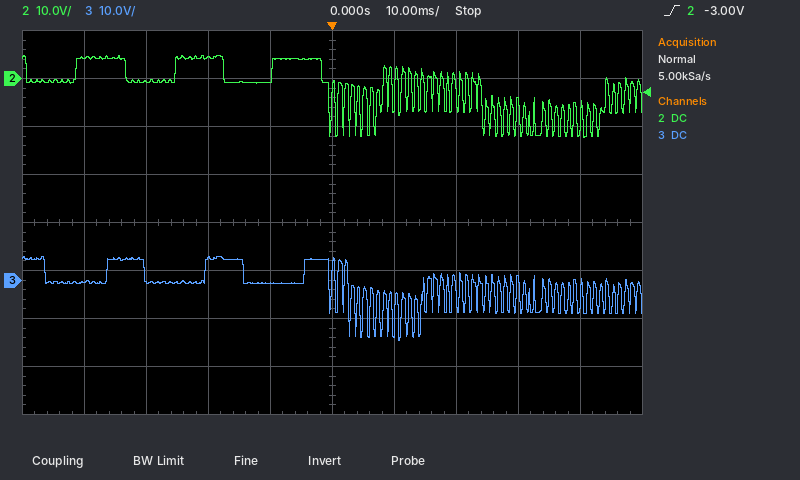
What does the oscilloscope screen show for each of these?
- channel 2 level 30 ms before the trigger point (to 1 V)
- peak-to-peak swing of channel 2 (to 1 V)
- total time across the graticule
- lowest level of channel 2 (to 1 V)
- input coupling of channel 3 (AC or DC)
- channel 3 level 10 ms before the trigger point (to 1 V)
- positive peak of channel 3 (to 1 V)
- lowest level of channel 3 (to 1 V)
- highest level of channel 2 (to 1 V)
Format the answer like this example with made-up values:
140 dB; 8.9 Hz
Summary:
-1 V; 17 V; 100 ms; -12 V; DC; -1 V; 5 V; -13 V; 5 V
